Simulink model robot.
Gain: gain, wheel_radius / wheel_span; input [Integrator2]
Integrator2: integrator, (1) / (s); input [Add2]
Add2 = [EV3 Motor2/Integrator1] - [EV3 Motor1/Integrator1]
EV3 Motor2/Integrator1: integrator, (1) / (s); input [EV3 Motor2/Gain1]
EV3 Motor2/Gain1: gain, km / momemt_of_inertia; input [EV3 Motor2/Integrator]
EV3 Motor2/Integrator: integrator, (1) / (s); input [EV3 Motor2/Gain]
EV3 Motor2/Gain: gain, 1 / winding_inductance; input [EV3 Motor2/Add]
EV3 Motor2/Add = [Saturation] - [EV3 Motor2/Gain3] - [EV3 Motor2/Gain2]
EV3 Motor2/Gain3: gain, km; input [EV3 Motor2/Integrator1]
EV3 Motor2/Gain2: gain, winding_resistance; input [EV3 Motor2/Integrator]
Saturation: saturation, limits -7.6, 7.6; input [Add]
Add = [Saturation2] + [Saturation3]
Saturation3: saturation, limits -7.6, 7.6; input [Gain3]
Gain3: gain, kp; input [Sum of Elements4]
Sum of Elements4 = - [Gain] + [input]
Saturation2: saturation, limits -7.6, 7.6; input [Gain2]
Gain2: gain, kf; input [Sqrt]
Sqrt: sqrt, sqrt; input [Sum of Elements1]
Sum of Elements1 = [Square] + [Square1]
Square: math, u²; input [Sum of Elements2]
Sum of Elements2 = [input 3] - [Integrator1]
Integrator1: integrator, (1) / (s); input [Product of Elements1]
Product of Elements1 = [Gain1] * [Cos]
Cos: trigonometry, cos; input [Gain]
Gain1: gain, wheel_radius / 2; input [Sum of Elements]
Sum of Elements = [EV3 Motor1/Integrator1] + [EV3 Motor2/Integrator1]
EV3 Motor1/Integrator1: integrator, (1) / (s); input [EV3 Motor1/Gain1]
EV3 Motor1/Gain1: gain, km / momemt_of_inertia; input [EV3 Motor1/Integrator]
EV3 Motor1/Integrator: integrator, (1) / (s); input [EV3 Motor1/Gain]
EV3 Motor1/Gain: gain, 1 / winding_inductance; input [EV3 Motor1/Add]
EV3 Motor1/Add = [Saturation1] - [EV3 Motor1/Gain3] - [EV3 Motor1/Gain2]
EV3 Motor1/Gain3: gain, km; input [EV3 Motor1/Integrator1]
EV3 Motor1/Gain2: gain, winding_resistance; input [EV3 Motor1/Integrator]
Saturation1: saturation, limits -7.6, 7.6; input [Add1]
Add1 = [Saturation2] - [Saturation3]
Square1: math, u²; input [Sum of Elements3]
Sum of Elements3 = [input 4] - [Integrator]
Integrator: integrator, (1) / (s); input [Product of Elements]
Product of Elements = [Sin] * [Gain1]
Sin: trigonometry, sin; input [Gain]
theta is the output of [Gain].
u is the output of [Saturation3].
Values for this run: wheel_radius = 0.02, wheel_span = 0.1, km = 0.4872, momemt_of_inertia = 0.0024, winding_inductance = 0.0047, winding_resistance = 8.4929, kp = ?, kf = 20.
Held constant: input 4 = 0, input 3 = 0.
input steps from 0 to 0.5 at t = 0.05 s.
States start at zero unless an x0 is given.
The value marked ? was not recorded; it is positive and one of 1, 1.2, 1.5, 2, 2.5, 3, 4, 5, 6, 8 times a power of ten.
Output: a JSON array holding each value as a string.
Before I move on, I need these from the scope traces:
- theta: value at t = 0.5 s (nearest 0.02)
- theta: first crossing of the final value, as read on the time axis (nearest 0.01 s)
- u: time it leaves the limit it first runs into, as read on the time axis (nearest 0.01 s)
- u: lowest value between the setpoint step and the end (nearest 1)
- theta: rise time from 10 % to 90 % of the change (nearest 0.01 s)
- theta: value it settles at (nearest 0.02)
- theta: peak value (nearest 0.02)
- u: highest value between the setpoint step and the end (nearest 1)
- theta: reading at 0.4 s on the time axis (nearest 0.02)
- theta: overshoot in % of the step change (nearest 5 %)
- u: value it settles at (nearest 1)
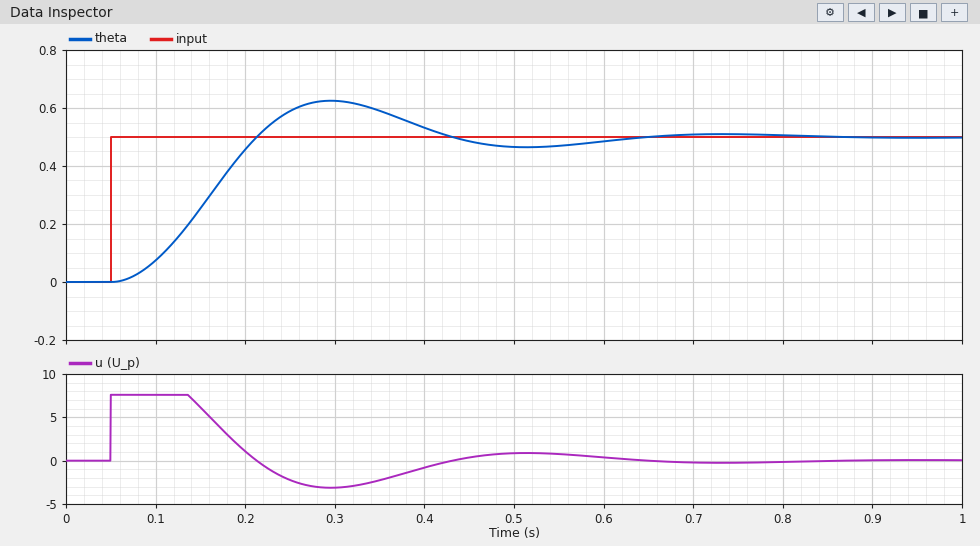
["0.46", "0.21 s", "0.14 s", "-3", "0.11 s", "0.50", "0.62", "8", "0.54", "25 %", "0"]
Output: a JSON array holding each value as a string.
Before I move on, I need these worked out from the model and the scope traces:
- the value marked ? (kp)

["25"]
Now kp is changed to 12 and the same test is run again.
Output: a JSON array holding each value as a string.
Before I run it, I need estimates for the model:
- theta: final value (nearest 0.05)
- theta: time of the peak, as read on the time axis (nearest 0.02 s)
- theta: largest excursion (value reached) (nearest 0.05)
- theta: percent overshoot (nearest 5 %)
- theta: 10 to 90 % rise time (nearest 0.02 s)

["0.50", "0.40 s", "0.55", "15 %", "0.16 s"]
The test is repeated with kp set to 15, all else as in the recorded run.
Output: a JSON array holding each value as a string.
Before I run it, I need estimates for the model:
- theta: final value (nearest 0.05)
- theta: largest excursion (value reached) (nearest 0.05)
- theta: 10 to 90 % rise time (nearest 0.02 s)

["0.50", "0.60", "0.14 s"]
